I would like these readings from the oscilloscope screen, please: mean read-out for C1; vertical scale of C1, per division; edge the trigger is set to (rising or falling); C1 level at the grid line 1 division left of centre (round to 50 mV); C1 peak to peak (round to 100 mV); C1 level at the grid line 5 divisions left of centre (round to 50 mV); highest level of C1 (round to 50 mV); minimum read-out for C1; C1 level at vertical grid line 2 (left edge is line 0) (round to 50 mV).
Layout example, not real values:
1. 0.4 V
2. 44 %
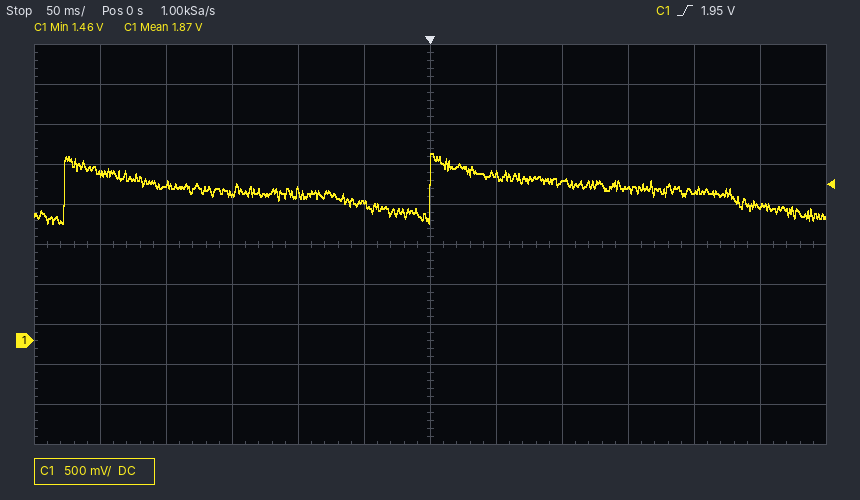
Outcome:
1. 1.87 V
2. 500 mV
3. rising
4. 1.70 V
5. 900 mV
6. 2.10 V
7. 2.35 V
8. 1.46 V
9. 1.95 V
